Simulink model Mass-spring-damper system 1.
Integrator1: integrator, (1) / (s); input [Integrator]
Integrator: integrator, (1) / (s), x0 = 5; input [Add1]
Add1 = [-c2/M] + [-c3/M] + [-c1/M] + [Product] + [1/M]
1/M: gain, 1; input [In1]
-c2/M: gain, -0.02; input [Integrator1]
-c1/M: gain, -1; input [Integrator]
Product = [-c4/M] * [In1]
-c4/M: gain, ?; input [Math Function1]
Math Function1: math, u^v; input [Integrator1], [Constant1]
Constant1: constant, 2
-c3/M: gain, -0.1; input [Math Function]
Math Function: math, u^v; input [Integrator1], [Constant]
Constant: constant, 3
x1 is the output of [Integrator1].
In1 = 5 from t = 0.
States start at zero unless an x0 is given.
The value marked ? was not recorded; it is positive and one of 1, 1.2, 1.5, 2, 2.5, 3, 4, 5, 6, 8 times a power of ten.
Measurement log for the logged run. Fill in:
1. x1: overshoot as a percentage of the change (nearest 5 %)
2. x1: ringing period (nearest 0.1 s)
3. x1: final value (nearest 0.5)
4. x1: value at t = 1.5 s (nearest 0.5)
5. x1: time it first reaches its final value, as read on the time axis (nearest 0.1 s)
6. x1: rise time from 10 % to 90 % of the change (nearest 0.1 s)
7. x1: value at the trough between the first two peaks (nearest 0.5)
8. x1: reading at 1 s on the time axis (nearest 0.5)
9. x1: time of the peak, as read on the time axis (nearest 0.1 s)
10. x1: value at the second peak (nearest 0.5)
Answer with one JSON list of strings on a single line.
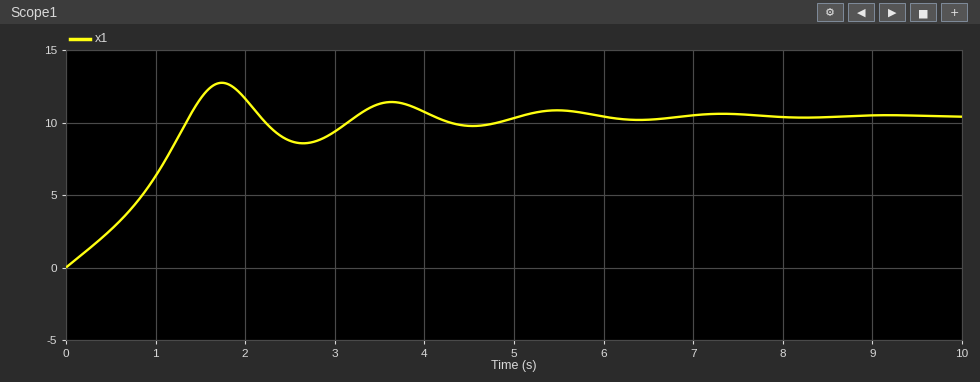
["20 %", "1.9 s", "10.5", "11.5", "1.4 s", "1.1 s", "8.5", "6.5", "1.7 s", "11.5"]
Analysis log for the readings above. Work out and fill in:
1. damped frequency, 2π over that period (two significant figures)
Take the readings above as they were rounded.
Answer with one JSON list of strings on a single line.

["3.3 rad/s"]
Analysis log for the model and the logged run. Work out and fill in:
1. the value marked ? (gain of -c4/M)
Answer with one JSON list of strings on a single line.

["0.2"]
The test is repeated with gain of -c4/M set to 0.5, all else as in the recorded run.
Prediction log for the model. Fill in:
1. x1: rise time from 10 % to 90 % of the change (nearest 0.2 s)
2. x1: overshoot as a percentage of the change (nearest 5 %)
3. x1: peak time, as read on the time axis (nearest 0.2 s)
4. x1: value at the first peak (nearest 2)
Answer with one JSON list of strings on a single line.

["0.8 s", "25 %", "1.4 s", "32"]
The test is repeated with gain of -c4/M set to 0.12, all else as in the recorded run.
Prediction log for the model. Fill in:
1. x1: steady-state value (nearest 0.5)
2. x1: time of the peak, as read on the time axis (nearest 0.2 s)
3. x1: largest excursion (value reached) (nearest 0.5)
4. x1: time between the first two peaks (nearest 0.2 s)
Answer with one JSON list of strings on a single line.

["7.0", "1.8 s", "8.5", "2.6 s"]
